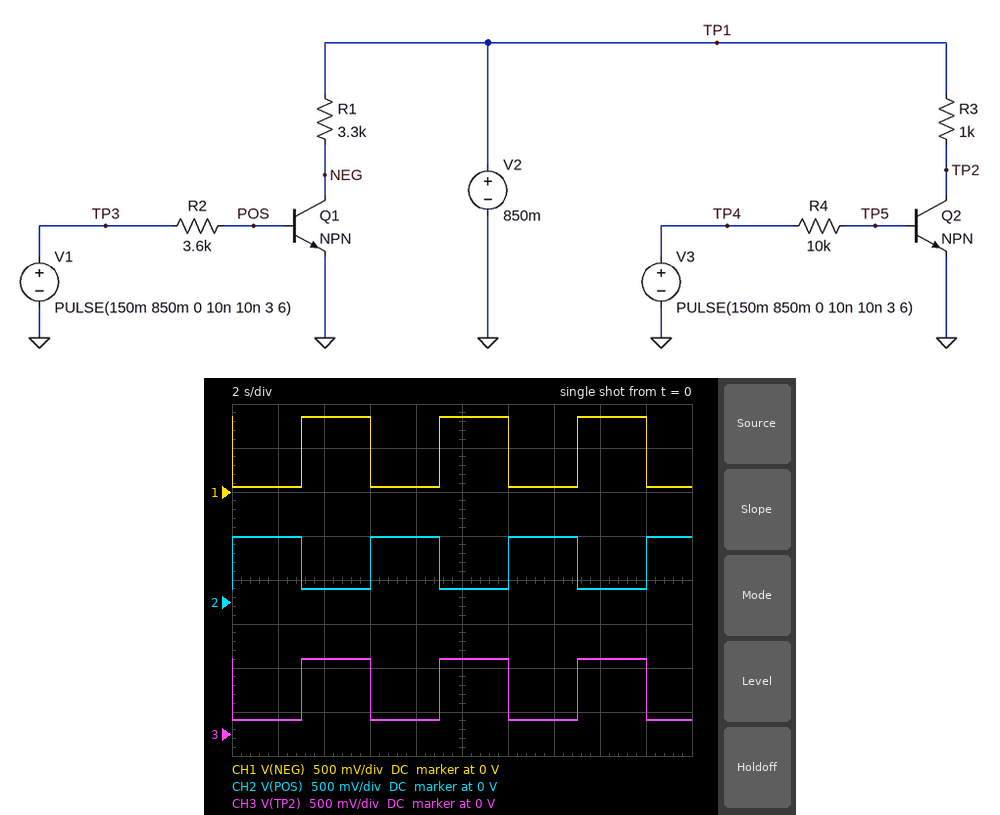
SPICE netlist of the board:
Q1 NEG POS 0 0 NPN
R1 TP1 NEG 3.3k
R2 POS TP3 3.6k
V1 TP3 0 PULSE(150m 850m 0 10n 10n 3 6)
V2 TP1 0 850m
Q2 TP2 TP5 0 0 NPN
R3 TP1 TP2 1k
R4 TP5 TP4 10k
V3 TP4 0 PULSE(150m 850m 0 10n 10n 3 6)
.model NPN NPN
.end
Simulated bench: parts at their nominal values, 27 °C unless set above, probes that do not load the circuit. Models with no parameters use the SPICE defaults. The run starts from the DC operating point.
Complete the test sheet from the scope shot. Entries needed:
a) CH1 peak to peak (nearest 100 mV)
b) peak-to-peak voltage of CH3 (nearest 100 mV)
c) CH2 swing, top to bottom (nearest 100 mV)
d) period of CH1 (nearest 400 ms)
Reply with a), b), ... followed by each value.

a) 800 mV
b) 700 mV
c) 600 mV
d) 6.0 s
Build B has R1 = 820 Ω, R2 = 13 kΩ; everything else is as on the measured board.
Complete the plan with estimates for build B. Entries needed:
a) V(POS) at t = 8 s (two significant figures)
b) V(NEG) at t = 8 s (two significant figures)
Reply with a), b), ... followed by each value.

a) 760 mV
b) 310 mV
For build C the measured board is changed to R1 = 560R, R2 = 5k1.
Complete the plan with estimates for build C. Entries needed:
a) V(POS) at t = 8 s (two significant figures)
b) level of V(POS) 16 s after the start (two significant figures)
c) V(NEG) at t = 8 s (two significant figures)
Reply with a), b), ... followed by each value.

a) 780 mV
b) 150 mV
c) 170 mV
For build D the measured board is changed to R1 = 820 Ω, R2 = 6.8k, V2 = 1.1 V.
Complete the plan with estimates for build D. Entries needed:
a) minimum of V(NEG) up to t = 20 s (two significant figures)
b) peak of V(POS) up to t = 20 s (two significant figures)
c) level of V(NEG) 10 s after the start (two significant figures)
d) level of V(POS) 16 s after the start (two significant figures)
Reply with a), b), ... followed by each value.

a) 220 mV
b) 780 mV
c) 1.1 V
d) 150 mV
